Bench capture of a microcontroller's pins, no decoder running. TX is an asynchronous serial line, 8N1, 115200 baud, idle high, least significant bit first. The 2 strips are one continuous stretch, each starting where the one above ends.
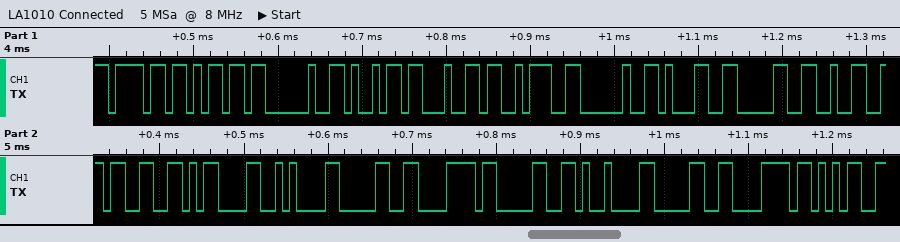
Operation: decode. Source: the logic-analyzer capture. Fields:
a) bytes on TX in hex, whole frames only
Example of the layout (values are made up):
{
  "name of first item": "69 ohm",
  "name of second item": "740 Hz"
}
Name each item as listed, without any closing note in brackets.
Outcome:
{
  "bytes on TX in hex, whole frames only": "0x6F 0x6D 0x20 0x69 0x64 0x3A 0x20 0x31 0x30 0x32 0x33 0x0D 0x0A 0x30 0x78 0x30 0x09 0x30 0x78 0x35"
}
